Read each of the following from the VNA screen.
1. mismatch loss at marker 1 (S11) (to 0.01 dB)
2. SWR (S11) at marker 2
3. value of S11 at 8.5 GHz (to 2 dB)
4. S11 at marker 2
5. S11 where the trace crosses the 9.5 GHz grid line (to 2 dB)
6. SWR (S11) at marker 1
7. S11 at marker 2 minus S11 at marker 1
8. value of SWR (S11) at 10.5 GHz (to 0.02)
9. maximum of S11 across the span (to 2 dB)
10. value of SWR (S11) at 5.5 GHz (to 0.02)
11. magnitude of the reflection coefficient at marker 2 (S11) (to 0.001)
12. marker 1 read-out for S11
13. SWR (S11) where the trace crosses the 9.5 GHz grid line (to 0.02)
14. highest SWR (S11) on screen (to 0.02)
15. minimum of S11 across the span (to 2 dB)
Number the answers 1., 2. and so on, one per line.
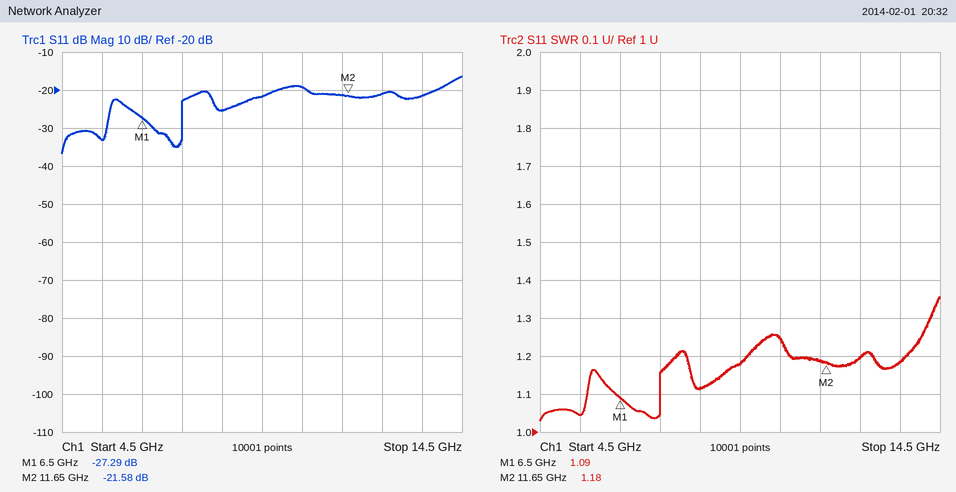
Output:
1. 0.01 dB
2. 1.18
3. -26 dB
4. -21.58 dB
5. -22 dB
6. 1.09
7. 5.71 dB
8. 1.24
9. -16 dB
10. 1.04
11. 0.083
12. -27.29 dB
13. 1.18
14. 1.36
15. -36 dB
